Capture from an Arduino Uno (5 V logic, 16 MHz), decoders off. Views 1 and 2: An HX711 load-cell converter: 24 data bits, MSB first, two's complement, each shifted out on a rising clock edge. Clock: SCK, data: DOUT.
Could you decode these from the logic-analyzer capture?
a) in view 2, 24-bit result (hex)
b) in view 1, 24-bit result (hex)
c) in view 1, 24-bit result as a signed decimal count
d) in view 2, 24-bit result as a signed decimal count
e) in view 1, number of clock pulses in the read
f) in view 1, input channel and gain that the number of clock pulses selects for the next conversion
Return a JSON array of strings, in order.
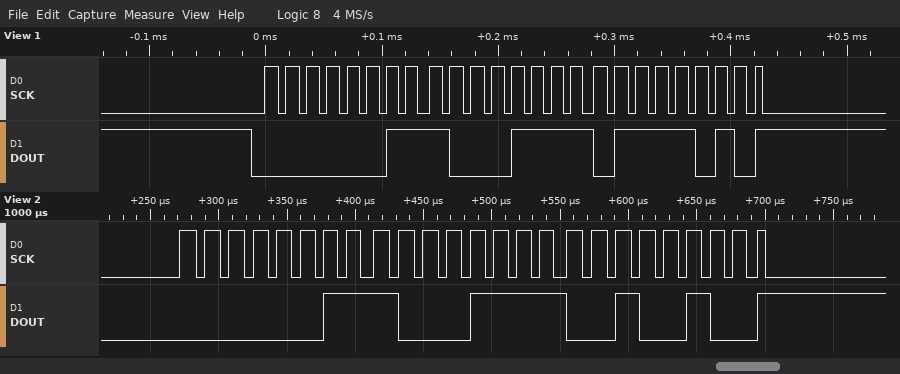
["0x038F24", "0x038F7A", "233338", "233252", "25", "channel A, gain 128"]
